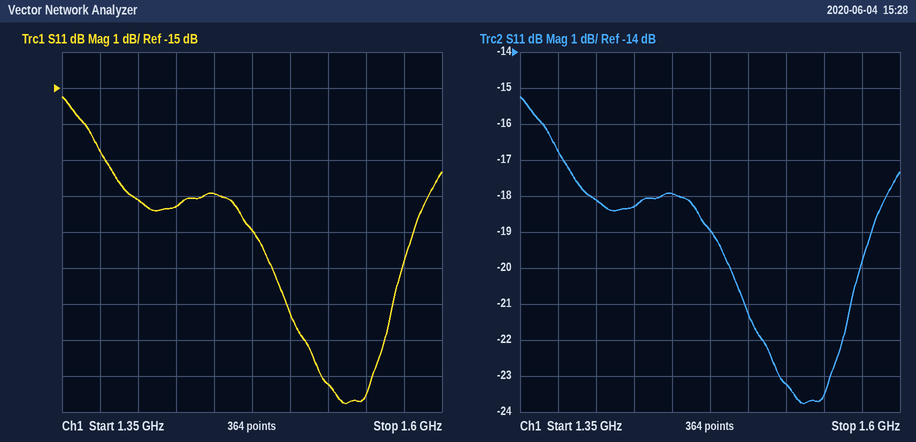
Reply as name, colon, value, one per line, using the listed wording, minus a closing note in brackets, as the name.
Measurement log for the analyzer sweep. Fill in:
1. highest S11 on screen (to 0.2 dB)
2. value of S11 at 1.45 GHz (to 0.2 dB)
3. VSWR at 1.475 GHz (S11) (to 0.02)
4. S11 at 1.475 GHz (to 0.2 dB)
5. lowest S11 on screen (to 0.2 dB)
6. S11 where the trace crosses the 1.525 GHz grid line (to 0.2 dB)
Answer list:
highest S11 on screen: -15.2 dB
value of S11 at 1.45 GHz: -18.0 dB
VSWR at 1.475 GHz (S11): 1.26
S11 at 1.475 GHz: -19.0 dB
lowest S11 on screen: -23.8 dB
S11 where the trace crosses the 1.525 GHz grid line: -23.2 dB
